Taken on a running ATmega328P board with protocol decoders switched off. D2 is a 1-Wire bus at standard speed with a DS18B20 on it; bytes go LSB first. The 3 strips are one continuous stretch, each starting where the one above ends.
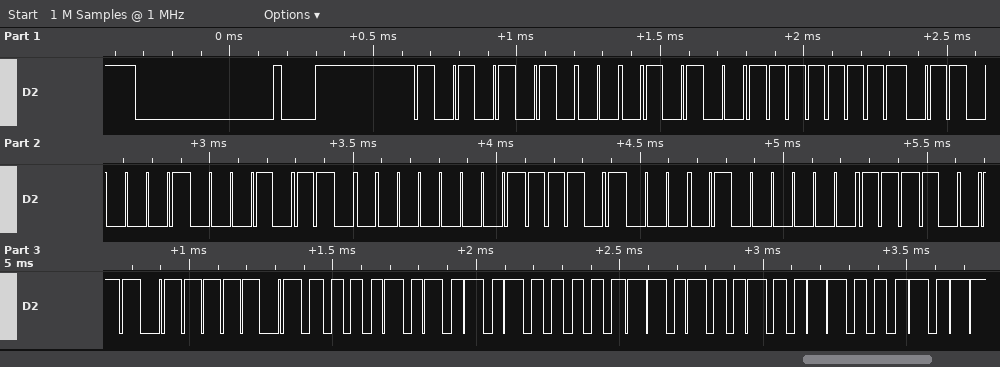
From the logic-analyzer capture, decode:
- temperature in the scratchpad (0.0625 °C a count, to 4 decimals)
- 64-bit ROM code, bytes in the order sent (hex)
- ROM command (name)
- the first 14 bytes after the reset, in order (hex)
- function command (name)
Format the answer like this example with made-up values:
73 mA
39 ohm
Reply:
85.0000 °C
28 FF 86 68 80 17 02 CF
Match ROM
55 28 FF 86 68 80 17 02 CF BE 50 05 4B 46
Read Scratchpad
